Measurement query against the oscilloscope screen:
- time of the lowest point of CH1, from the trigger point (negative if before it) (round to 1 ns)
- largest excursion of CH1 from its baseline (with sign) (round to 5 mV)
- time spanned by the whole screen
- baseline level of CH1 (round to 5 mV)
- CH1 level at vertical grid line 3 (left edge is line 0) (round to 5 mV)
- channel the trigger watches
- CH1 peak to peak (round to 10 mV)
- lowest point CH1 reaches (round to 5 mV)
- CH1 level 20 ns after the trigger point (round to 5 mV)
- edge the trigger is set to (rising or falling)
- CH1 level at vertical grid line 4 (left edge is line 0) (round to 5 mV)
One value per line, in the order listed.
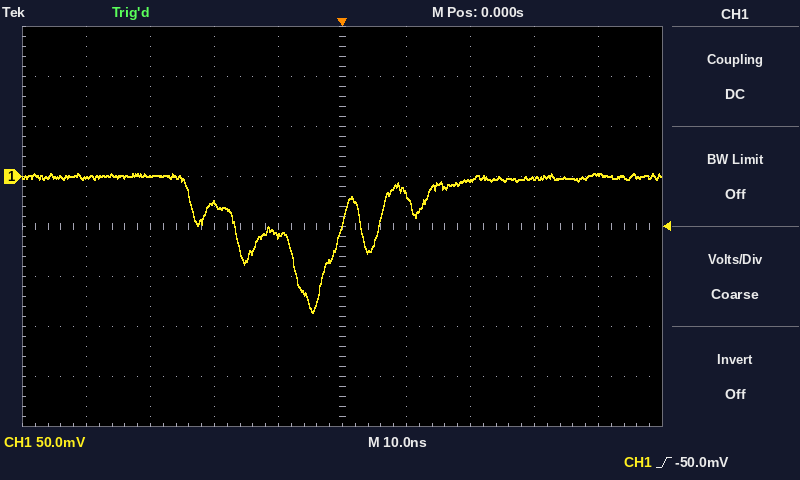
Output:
-5 ns
-135 mV
100 ns
0 mV
-25 mV
CH1
140 mV
-135 mV
-5 mV
rising
-60 mV
